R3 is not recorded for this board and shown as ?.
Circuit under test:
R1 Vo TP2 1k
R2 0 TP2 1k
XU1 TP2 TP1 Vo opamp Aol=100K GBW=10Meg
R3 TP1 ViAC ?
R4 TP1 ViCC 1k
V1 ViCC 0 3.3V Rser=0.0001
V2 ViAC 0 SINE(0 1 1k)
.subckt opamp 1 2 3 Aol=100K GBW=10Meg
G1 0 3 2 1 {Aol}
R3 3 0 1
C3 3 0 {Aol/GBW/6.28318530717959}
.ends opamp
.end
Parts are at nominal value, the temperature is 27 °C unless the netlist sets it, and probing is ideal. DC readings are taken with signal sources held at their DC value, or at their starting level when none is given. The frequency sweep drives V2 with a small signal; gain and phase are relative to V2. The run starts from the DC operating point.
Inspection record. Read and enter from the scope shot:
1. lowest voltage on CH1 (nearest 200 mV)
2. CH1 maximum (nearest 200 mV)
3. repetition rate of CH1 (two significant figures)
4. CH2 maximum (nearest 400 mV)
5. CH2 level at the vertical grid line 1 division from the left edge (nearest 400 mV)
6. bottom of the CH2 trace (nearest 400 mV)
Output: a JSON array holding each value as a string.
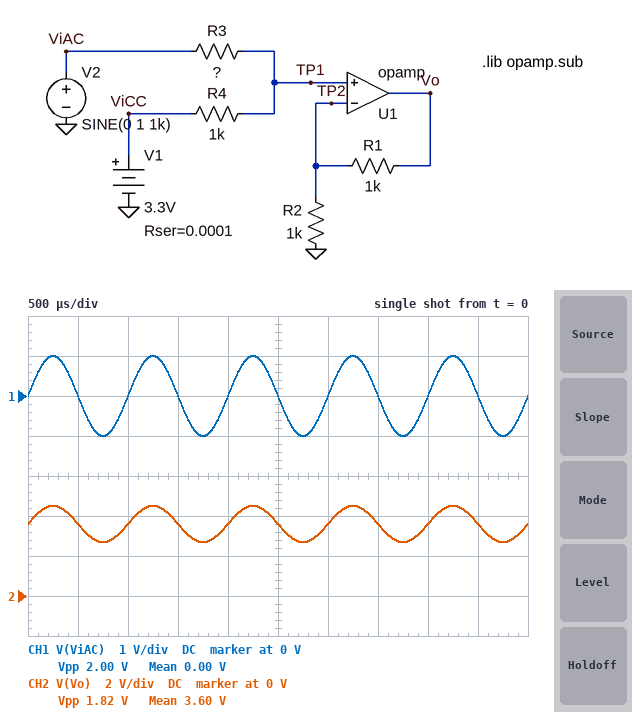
["-1.0 V", "1.0 V", "1.0 kHz", "4.4 V", "3.6 V", "2.8 V"]
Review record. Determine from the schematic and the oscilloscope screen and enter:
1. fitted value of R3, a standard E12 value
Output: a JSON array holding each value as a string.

["1.2 kΩ"]
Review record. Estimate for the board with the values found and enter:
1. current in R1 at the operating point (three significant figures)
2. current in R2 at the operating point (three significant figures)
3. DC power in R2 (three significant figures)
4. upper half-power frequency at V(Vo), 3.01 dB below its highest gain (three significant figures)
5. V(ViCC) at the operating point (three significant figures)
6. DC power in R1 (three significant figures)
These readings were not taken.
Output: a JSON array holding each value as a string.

["1.80 mA", "1.80 mA", "3.24 mW", "5.00 MHz", "3.30 V", "3.24 mW"]
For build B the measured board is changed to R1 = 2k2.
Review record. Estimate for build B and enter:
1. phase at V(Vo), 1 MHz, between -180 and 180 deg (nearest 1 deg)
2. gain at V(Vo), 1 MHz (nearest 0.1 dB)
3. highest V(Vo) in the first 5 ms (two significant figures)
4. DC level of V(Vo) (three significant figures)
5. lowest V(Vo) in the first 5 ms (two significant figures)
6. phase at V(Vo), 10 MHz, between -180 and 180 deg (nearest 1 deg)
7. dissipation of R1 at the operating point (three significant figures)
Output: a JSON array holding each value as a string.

["-18 deg", "2.8 dB", "7.2 V", "5.76 V", "4.3 V", "-73 deg", "7.13 mW"]
